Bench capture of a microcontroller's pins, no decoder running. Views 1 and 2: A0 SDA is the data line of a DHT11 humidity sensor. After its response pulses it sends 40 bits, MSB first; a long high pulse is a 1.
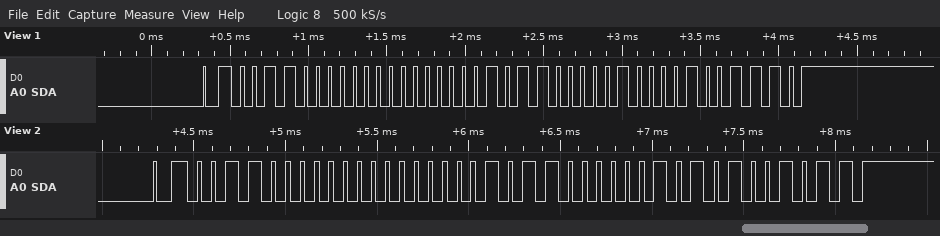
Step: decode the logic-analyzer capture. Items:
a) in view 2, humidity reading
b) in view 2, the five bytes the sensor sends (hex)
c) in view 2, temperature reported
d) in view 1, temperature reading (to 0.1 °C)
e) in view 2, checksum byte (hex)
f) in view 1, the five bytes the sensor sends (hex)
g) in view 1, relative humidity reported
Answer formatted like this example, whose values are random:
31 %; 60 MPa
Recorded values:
48 %; 30 00 16 05 4B; 22.5 °C; 22.8 °C; 0x4B; 30 00 16 08 4E; 48 %
